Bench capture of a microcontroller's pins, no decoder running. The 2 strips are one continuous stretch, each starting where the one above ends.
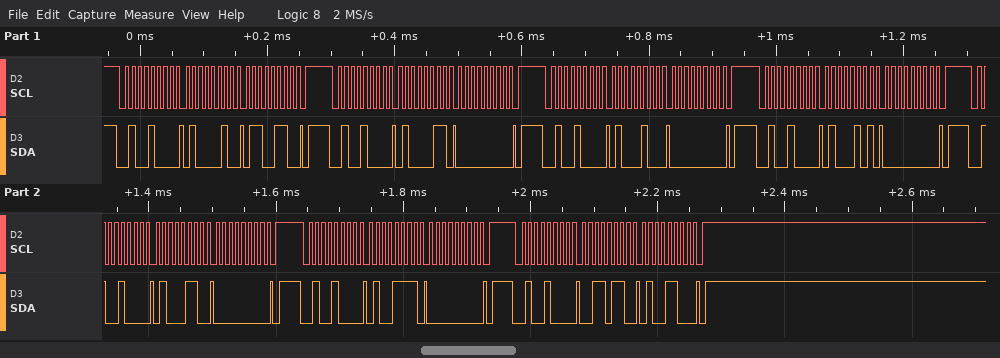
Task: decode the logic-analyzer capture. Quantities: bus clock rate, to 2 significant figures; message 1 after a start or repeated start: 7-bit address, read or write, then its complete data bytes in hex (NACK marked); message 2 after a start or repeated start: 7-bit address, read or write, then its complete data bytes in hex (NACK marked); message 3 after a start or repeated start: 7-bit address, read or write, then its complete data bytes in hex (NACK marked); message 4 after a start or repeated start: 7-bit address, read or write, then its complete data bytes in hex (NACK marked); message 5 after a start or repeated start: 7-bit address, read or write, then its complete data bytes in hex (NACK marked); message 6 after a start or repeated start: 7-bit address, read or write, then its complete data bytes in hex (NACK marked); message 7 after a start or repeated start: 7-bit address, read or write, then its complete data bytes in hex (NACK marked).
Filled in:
100 kHz
0x24 write: 42 66
0x24 write: 43 00
0x24 write: 44 00
0x24 write: 45 00
0x24 write: 46 00
0x24 write: 4F 00
0x24 write: 36 4C
